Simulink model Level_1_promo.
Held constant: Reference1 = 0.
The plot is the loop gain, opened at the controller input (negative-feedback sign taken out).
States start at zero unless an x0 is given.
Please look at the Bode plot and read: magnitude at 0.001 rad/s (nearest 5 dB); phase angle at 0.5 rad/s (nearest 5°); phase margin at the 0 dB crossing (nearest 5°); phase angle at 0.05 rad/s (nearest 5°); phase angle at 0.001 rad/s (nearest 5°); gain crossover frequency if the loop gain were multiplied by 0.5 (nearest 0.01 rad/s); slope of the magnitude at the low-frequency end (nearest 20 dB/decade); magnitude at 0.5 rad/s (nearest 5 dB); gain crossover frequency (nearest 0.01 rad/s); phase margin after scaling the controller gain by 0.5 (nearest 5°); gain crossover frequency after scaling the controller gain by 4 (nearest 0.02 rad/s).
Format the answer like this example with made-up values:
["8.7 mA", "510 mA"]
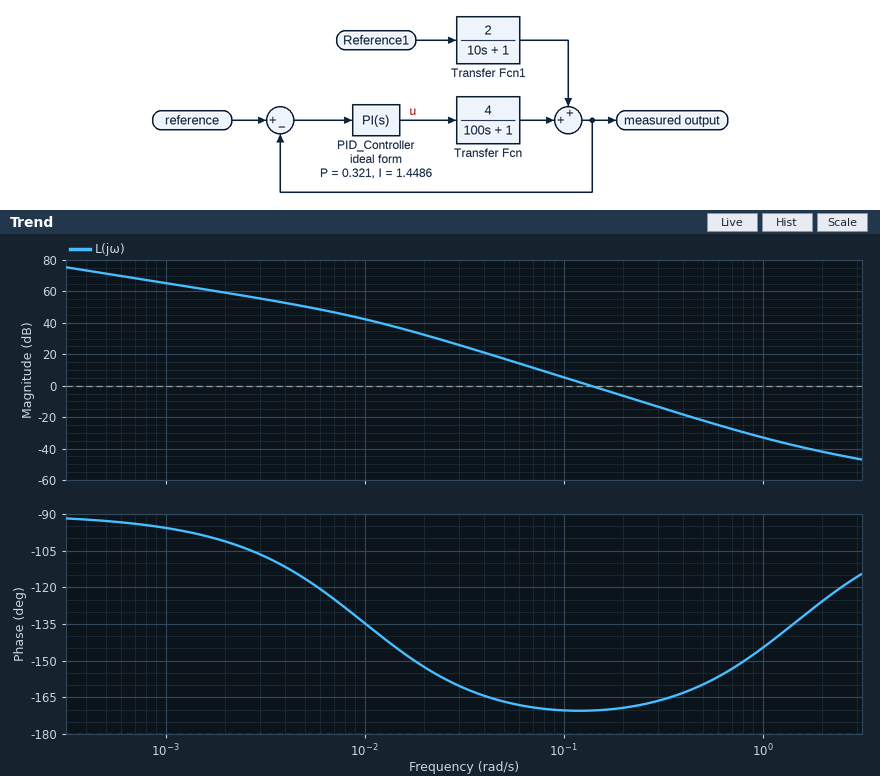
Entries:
["65 dB", "-160°", "10°", "-165°", "-95°", "0.10 rad/s", "-20 dB/decade", "-20 dB", "0.14 rad/s", "10°", "0.28 rad/s"]
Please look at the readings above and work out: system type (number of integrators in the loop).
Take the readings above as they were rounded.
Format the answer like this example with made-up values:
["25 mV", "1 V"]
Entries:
["1"]
